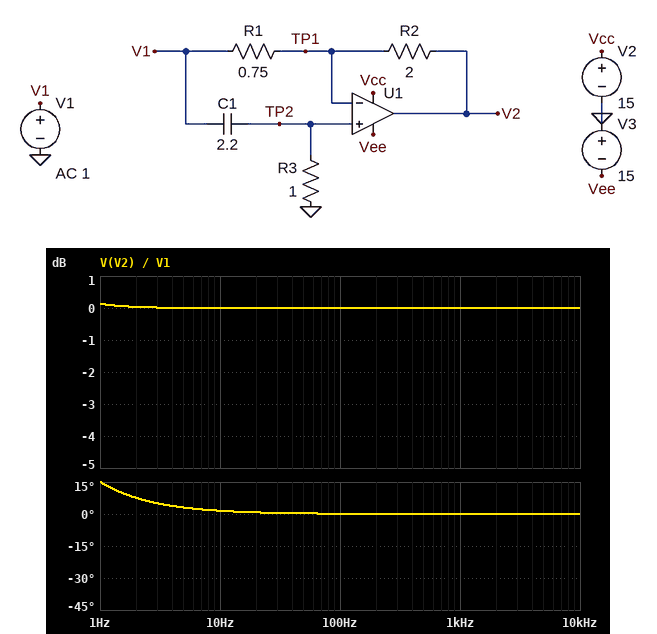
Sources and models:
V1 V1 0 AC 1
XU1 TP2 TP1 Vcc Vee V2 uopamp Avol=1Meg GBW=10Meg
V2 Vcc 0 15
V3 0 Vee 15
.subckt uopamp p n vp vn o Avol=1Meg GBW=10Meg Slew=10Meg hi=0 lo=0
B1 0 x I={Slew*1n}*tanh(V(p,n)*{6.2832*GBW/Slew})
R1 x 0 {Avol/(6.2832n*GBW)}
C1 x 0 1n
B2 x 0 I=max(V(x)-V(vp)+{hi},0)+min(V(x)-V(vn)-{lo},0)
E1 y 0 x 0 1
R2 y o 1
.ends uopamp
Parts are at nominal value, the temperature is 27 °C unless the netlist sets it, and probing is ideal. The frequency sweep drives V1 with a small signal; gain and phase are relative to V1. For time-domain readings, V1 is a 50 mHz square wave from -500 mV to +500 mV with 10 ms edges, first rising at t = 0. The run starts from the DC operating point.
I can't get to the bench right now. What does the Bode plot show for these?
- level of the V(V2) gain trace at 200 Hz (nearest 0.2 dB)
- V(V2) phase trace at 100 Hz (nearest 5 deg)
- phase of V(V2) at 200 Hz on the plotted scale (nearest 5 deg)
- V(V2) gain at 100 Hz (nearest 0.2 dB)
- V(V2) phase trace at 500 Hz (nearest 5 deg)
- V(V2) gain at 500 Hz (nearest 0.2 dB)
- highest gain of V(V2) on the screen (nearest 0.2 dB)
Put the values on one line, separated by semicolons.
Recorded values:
0 dB; 0 deg; 0 deg; 0 dB; 0 deg; 0 dB; 0.2 dB
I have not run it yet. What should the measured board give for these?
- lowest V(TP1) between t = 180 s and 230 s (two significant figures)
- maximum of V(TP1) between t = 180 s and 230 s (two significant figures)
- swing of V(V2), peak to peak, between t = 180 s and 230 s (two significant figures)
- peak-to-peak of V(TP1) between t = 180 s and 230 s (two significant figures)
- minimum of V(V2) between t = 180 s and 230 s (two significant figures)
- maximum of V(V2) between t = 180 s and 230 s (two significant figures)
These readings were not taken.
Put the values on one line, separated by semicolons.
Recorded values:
-990 mV; 990 mV; 4.6 V; 2.0 V; -2.3 V; 2.3 V
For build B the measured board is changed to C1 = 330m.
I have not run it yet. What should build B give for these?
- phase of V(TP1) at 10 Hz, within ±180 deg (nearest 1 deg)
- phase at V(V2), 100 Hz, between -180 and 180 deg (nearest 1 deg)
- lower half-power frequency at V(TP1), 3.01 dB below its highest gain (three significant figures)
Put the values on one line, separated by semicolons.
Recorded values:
3 deg; 1 deg; 482 mHz
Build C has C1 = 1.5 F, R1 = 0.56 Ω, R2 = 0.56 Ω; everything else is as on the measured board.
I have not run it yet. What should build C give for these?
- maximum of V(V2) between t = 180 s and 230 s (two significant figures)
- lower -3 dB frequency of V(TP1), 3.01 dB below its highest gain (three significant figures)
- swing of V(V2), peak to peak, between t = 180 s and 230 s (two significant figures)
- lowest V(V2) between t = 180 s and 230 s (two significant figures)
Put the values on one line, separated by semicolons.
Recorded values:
1.5 V; 106 mHz; 3.0 V; -1.5 V
